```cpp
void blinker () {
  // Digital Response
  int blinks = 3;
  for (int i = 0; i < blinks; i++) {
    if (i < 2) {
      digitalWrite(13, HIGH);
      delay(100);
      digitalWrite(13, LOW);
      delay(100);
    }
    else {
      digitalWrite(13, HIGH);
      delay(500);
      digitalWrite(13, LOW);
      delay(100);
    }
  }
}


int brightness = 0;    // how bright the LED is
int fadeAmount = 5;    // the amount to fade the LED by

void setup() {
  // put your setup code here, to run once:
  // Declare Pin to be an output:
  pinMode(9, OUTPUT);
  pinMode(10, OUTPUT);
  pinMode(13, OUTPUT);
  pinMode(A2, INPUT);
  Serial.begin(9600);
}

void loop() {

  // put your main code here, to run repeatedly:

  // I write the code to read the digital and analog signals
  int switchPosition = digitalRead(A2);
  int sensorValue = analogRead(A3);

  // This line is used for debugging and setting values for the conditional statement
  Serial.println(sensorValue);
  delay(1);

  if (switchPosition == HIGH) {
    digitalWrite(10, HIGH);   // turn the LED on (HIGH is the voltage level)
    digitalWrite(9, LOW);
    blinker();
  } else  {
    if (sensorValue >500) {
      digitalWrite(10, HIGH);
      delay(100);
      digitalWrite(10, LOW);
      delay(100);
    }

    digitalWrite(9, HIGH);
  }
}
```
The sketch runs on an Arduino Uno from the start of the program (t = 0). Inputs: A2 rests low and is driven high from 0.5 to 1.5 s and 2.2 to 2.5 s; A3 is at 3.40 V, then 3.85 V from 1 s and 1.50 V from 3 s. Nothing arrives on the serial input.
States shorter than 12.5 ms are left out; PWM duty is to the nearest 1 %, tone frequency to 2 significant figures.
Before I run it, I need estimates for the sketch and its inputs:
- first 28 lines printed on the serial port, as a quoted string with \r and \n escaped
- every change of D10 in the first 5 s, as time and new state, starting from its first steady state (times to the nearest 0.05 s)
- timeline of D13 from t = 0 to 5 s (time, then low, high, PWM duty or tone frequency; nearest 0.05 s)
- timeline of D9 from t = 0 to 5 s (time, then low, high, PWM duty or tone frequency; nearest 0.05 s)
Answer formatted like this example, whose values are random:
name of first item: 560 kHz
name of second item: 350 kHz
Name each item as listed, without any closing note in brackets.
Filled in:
first 28 lines printed on the serial port, as a quoted string with \r and \n escaped: "696\r\n696\r\n696\r\n696\r\n788\r\n788\r\n788\r\n788\r\n307\r\n307\r\n307\r\n307\r\n307\r\n307\r\n307\r\n307\r\n307\r\n307\r\n307\r\n307\r\n307\r\n307\r\n307\r\n307\r\n307\r\n307\r\n307\r\n307\r\n"
every change of D10 in the first 5 s, as time and new state, starting from its first steady state: 0 s high; 0.1 s low; 0.2 s high; 0.3 s low; 0.4 s high; 0.5 s low; 0.6 s high; 1.7 s low; 1.8 s high; 1.9 s low; 2 s high; 2.1 s low; 2.2 s high
timeline of D13 from t = 0 to 5 s: 0 s low; 0.6 s high; 0.7 s low; 0.8 s high; 0.9 s low; 1 s high; 1.5 s low; 2.2 s high; 2.3 s low; 2.4 s high; 2.5 s low; 2.6 s high; 3.1 s low
timeline of D9 from t = 0 to 5 s: 0 s low; 0.2 s high; 0.6 s low; 1.8 s high; 2.2 s low; 3.2 s high
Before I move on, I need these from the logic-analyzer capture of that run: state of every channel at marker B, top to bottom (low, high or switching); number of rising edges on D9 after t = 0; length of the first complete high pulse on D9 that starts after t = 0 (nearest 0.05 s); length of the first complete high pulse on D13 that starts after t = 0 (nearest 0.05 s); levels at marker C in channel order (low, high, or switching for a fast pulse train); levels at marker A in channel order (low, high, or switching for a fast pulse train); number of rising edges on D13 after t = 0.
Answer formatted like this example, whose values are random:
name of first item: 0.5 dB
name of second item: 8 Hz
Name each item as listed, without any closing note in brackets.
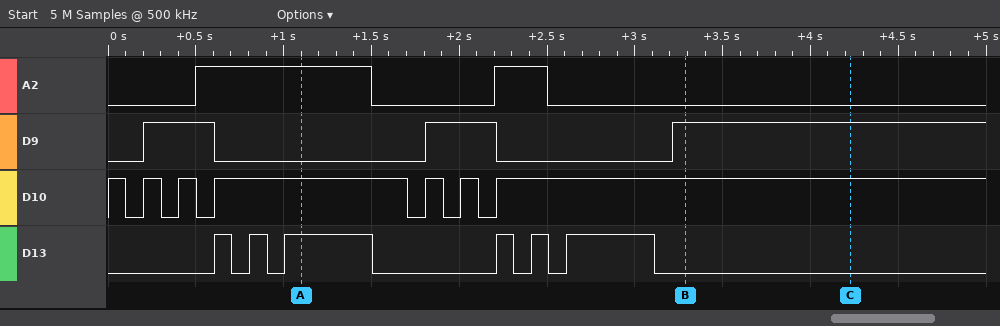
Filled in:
state of every channel at marker B, top to bottom: A2 low, D9 high, D10 high, D13 low
number of rising edges on D9 after t = 0: 3
length of the first complete high pulse on D9 that starts after t = 0: 0.40 s
length of the first complete high pulse on D13 that starts after t = 0: 0.10 s
levels at marker C in channel order: A2 low, D9 high, D10 high, D13 low
levels at marker A in channel order: A2 high, D9 low, D10 high, D13 high
number of rising edges on D13 after t = 0: 6
